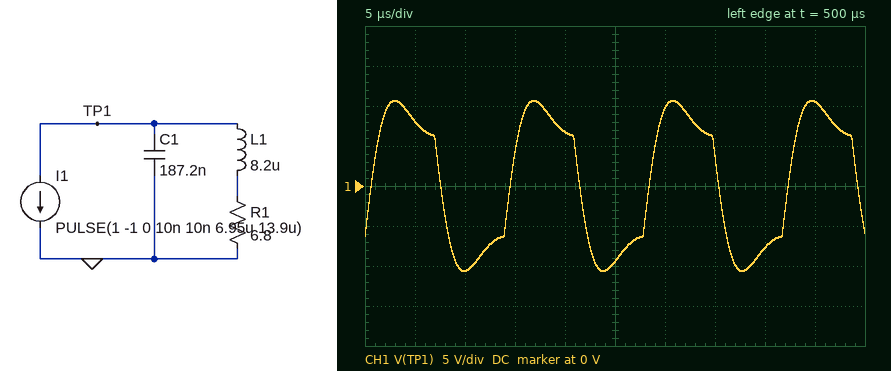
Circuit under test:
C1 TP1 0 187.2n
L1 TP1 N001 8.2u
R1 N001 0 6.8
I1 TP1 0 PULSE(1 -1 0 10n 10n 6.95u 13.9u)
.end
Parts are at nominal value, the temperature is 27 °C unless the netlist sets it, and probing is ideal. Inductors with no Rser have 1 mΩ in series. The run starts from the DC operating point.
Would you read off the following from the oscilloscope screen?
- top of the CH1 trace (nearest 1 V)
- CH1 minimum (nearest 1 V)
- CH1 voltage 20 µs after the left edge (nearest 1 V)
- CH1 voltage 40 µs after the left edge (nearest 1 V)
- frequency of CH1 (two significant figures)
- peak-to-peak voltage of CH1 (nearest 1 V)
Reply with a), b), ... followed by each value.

a) 11 V
b) -11 V
c) 7 V
d) -8 V
e) 72 kHz
f) 21 V
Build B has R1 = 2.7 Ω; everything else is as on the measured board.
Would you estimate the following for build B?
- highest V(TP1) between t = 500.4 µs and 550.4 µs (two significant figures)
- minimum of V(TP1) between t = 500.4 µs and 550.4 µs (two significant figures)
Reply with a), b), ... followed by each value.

a) 10 V
b) -10 V
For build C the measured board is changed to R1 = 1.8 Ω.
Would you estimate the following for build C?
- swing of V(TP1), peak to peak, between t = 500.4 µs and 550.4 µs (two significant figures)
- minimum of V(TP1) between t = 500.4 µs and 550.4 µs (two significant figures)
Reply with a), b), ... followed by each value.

a) 19 V
b) -9.6 V
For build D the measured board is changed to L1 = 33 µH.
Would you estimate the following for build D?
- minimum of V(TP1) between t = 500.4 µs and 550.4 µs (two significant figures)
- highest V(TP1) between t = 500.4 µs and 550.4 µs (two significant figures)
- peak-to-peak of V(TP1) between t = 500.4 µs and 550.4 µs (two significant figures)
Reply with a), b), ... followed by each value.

a) -32 V
b) 32 V
c) 64 V
